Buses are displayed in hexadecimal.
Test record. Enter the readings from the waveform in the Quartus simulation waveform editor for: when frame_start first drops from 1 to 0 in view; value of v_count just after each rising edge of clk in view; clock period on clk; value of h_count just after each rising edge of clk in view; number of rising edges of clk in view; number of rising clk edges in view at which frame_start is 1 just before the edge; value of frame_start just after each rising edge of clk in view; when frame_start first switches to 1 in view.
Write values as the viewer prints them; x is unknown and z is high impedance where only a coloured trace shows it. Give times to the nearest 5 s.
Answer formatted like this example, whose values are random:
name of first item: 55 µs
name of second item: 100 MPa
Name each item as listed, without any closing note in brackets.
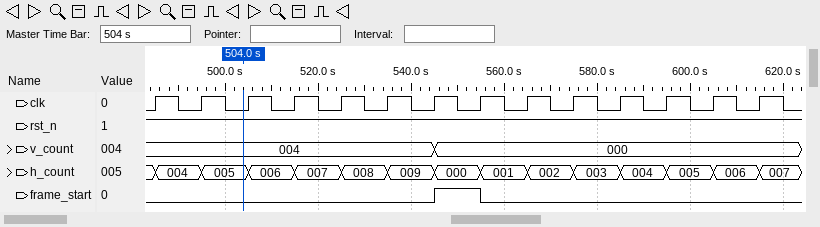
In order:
when frame_start first drops from 1 to 0 in view: 555 s
value of v_count just after each rising edge of clk in view: 004, 004, 004, 004, 004, 004, 000, 000, 000, 000, 000, 000, 000, 000
clock period on clk: 10 s
value of h_count just after each rising edge of clk in view: 004, 005, 006, 007, 008, 009, 000, 001, 002, 003, 004, 005, 006, 007
number of rising edges of clk in view: 14
number of rising clk edges in view at which frame_start is 1 just before the edge: 1
value of frame_start just after each rising edge of clk in view: 0 0 0 0 0 0 1 0 0 0 0 0 0 0
when frame_start first switches to 1 in view: 545 s
